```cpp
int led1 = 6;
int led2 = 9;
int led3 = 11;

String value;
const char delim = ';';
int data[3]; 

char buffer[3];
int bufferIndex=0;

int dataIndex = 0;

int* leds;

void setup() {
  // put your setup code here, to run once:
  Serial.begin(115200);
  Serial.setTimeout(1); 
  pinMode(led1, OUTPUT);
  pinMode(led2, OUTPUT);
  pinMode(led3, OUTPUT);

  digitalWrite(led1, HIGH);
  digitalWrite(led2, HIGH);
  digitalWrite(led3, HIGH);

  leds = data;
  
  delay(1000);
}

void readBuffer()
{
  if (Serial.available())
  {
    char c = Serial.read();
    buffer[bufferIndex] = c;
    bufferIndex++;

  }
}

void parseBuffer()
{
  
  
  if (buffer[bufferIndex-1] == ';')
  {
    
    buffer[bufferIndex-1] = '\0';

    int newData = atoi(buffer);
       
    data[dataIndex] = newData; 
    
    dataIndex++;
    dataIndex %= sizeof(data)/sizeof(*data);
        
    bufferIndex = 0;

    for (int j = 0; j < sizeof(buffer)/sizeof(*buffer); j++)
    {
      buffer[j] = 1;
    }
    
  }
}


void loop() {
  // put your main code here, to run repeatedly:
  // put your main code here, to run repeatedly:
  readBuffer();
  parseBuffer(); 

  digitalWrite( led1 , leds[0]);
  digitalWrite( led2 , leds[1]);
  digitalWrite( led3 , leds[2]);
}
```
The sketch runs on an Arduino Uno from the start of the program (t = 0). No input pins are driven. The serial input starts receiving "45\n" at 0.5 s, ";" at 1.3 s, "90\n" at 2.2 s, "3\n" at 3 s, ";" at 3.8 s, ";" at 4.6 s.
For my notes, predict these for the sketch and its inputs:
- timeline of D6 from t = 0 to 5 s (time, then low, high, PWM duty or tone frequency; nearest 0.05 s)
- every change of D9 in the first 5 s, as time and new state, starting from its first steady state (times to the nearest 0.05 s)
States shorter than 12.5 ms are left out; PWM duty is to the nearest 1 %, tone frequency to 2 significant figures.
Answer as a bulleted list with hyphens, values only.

- 0 s high; 1 s low; 1.3 s high
- 0 s high; 1 s low; 3.8 s high
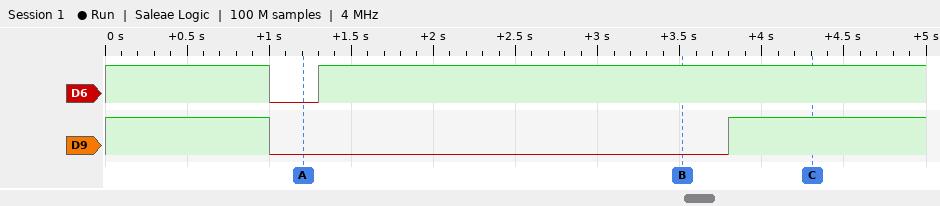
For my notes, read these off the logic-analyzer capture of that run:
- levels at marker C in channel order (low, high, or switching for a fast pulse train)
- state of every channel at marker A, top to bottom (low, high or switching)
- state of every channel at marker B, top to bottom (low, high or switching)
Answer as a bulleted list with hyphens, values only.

- D6 high, D9 high
- D6 low, D9 low
- D6 high, D9 low
